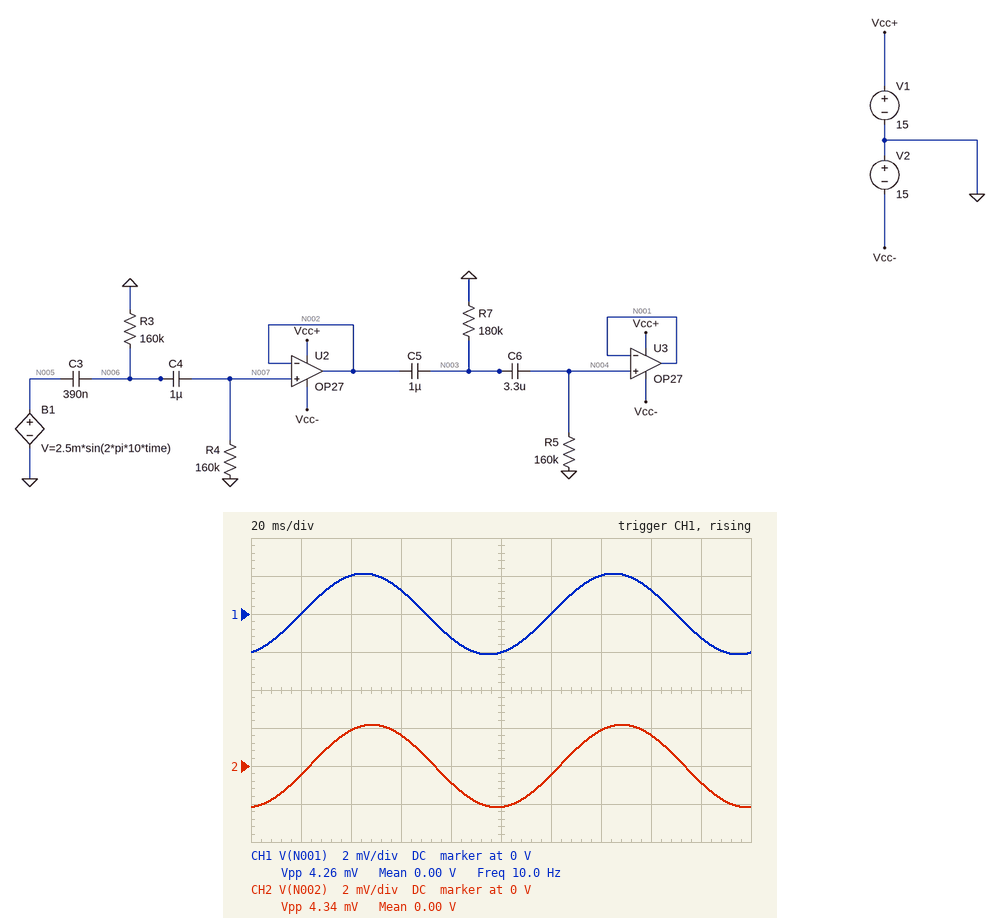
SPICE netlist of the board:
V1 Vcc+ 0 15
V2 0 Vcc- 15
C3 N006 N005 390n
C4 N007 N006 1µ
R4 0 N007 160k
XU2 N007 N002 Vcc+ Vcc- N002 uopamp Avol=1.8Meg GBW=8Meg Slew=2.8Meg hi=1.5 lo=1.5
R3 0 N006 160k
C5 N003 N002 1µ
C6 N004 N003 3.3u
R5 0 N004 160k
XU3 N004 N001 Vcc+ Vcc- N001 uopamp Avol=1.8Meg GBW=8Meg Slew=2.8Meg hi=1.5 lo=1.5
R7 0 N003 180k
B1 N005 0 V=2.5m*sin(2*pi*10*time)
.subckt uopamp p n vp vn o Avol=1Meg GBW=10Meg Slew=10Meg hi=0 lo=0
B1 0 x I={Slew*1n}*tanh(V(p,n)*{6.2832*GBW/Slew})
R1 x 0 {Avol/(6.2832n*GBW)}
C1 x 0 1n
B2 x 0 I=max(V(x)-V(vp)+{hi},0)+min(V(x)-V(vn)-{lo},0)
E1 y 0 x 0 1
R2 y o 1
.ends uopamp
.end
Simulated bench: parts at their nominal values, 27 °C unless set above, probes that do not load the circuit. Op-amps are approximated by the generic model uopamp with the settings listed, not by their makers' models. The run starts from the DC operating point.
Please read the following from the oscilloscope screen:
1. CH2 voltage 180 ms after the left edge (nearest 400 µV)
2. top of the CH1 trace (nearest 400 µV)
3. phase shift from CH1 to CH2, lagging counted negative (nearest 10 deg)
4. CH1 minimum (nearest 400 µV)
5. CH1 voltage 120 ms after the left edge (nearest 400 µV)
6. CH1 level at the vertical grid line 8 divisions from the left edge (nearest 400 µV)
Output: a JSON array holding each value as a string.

["-800 µV", "2.0 mV", "-10 deg", "-2.0 mV", "0 V", "1.2 mV"]
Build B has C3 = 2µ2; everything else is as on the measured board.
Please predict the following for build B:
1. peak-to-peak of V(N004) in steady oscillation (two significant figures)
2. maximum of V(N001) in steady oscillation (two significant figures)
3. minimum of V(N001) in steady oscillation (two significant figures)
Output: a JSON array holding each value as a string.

["4.8 mV", "2.4 mV", "-2.4 mV"]
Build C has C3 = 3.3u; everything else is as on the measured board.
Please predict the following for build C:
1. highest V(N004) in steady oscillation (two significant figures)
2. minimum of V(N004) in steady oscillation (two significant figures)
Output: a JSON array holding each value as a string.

["2.4 mV", "-2.4 mV"]
